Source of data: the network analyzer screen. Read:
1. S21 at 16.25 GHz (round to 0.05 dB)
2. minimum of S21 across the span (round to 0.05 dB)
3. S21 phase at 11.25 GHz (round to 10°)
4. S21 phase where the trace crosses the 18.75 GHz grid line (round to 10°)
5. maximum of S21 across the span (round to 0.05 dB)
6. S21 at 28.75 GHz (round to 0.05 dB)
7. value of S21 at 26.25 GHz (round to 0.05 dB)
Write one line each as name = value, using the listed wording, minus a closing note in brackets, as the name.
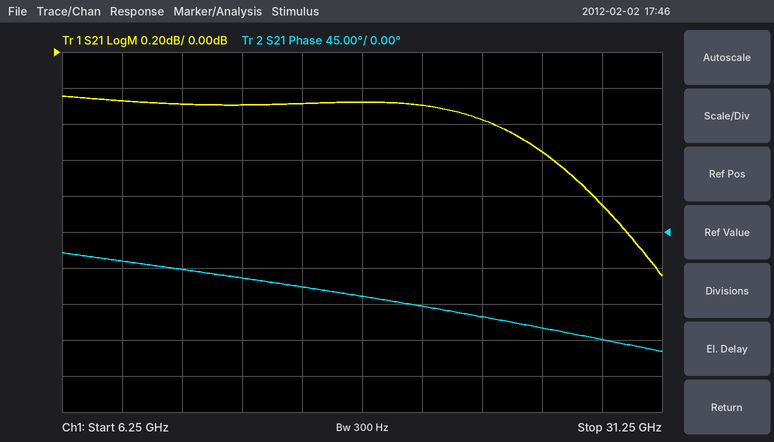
S21 at 16.25 GHz = -0.30 dB
minimum of S21 across the span = -1.25 dB
S21 phase at 11.25 GHz = -50°
S21 phase where the trace crosses the 18.75 GHz grid line = -80°
maximum of S21 across the span = -0.25 dB
S21 at 28.75 GHz = -0.85 dB
value of S21 at 26.25 GHz = -0.55 dB
